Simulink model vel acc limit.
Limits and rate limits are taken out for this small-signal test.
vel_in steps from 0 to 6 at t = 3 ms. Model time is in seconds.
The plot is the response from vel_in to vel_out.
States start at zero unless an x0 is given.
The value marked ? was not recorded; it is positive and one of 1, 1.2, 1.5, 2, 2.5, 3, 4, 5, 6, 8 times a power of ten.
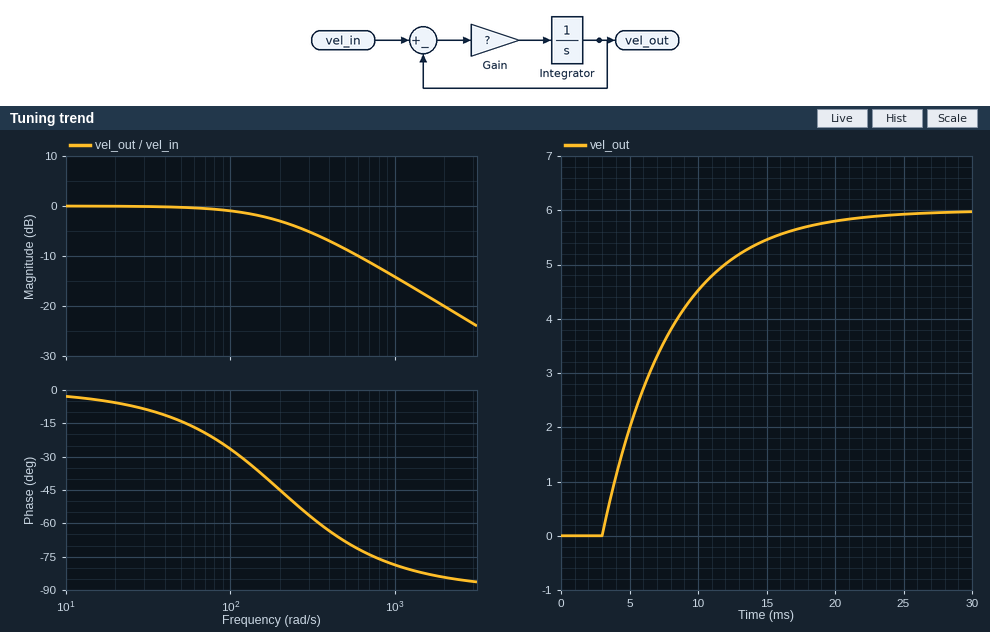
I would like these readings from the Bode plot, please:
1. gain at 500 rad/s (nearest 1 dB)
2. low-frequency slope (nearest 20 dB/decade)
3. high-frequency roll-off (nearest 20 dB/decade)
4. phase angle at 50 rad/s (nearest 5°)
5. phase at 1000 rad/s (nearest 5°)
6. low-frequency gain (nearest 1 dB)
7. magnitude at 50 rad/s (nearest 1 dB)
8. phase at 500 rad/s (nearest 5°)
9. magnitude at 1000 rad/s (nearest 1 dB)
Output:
-9 dB
0 dB/decade
-20 dB/decade
-15°
-80°
0 dB
0 dB
-70°
-14 dB
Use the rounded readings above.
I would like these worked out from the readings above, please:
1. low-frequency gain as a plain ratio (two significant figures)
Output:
1.0
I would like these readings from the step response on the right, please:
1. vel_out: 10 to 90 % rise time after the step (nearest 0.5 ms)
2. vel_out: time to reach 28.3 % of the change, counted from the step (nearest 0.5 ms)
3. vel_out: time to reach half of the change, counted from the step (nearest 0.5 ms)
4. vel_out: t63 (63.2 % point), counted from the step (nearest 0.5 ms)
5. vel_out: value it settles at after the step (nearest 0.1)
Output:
11.0 ms
1.5 ms
3.5 ms
5.0 ms
6.0
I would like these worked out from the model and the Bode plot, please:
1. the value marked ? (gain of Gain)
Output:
200
